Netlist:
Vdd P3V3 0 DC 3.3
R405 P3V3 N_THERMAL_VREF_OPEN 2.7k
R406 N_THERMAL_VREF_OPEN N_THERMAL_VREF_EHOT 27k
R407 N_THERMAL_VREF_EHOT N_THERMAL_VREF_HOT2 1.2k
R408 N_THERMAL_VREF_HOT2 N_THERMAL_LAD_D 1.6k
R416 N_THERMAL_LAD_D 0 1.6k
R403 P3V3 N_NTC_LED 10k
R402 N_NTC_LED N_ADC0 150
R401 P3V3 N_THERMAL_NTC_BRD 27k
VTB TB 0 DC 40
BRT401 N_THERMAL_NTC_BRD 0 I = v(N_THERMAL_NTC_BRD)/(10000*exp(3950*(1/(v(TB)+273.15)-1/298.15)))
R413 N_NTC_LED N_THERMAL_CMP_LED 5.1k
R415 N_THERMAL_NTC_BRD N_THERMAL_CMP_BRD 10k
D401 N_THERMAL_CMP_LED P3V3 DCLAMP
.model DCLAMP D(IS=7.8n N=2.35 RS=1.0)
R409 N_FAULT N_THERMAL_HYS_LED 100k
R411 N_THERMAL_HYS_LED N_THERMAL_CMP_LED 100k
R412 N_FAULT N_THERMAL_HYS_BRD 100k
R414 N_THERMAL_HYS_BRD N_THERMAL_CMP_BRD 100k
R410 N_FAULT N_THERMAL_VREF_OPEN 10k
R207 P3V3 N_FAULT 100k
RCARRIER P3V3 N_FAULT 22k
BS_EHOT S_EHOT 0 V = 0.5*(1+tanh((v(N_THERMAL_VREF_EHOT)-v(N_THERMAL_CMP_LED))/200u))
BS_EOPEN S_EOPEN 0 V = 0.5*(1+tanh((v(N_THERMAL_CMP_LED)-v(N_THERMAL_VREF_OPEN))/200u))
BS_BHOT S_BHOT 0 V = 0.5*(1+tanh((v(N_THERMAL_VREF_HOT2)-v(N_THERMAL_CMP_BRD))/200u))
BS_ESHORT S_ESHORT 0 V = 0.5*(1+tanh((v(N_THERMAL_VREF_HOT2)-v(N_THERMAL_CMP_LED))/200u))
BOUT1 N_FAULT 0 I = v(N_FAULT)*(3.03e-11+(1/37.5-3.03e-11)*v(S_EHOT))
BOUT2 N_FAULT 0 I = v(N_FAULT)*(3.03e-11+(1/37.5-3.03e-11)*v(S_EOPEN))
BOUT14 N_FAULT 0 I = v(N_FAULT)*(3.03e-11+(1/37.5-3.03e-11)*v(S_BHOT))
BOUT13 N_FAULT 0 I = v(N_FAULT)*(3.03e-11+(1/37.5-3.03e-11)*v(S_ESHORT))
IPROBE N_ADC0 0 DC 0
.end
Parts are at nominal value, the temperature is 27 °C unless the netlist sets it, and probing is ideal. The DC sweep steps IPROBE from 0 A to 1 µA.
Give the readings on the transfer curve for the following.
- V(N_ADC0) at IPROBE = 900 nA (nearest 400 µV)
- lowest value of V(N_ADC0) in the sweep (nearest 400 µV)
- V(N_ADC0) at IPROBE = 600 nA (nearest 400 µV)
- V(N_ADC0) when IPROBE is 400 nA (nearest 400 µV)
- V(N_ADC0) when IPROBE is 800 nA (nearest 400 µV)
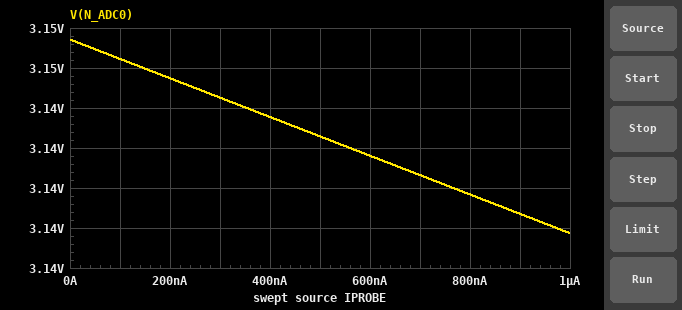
3.1388 V
3.1376 V
3.1416 V
3.1436 V
3.1396 V
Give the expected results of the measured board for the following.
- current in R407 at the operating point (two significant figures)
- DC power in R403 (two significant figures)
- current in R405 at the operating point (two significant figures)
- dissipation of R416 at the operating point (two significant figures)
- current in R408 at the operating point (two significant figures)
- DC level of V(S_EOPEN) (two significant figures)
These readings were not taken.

78 µA
2.3 µW
320 µA
9.6 µW
78 µA
1.0 V
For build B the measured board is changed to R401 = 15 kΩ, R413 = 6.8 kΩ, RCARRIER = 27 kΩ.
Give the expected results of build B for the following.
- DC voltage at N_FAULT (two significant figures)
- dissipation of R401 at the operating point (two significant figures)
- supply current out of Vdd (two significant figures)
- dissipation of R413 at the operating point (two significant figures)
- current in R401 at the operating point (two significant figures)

16 mV
400 µW
650 µA
1.6 µW
160 µA
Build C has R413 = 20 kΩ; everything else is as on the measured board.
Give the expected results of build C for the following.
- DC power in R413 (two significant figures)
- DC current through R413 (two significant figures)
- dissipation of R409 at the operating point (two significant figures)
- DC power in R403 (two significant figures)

4.1 µW
14 µA
20 µW
2.0 µW
